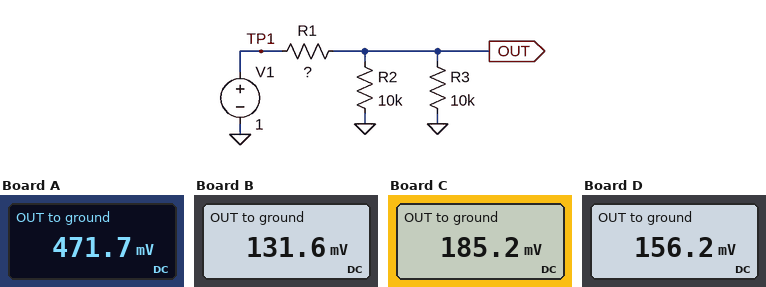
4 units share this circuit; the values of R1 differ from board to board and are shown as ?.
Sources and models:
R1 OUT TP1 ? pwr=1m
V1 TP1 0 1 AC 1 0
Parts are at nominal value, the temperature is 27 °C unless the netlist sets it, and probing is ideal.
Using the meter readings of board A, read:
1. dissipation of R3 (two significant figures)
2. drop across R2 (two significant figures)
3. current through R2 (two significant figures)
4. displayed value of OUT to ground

22 µW
470 mV
47 µA
471.7 mV
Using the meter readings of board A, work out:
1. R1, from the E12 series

5.6 kΩ
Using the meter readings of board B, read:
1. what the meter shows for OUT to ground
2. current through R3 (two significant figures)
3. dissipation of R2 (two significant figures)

131.6 mV
13 µA
1.7 µW
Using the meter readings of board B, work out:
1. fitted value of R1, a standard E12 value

33 kΩ
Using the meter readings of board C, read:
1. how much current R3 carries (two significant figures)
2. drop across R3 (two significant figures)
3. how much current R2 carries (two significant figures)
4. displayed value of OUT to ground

19 µA
190 mV
19 µA
185.2 mV
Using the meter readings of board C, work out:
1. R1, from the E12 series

22 kΩ
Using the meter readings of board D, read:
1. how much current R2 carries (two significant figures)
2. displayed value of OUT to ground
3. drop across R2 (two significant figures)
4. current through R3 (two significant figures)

16 µA
156.2 mV
160 mV
16 µA
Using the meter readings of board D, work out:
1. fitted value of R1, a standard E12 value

27 kΩ
